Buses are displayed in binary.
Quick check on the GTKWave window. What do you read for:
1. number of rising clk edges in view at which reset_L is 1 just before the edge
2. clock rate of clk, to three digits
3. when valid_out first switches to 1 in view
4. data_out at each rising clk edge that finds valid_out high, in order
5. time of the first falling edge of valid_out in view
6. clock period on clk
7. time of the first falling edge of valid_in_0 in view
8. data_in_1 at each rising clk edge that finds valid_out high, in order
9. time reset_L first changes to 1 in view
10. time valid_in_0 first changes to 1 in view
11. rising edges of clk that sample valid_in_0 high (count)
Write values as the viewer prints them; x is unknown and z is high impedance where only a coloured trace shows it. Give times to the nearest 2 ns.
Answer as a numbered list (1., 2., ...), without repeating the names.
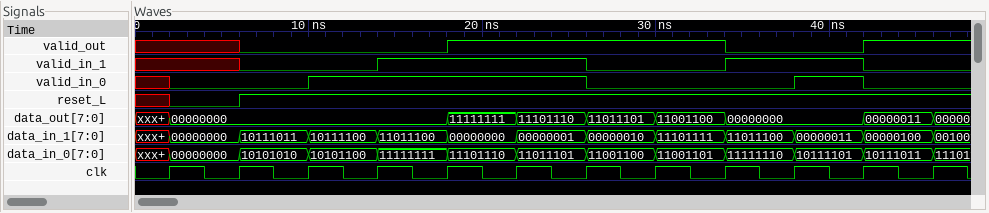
1. 10
2. 250 MHz
3. 18 ns
4. 11111111, 11101110, 11011101, 11001100, 00000011
5. 34 ns
6. 4 ns
7. 26 ns
8. 00000000, 00000001, 00000010, 11101111, 00000100
9. 6 ns
10. 10 ns
11. 5
